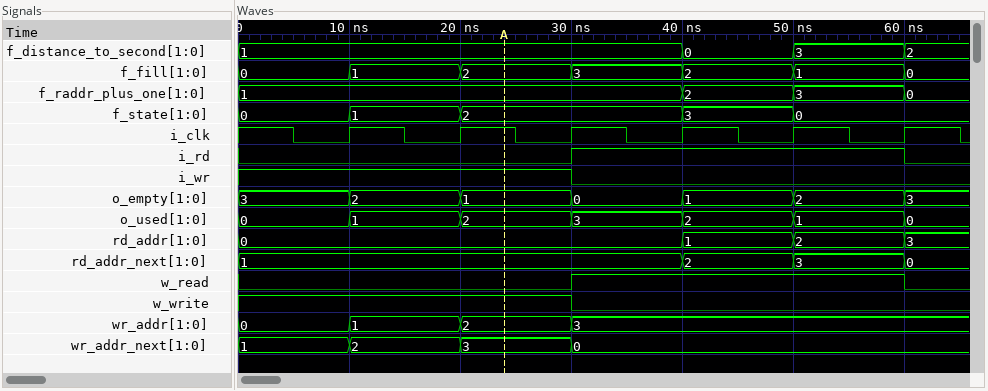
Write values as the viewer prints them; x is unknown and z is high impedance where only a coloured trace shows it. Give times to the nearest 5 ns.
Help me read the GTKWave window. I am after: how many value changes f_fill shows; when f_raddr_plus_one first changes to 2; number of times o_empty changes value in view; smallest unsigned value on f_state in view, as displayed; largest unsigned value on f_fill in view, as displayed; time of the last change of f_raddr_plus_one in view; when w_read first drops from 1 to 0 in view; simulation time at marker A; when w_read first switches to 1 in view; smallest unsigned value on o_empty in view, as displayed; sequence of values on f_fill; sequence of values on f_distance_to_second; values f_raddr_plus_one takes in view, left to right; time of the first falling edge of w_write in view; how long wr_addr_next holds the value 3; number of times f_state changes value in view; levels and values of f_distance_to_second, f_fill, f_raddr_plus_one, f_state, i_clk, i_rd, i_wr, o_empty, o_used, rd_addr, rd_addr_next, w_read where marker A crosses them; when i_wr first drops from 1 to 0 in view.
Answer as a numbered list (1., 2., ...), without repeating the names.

1. 6
2. 40 ns
3. 6
4. 0
5. 3
6. 60 ns
7. 60 ns
8. 25 ns
9. 30 ns
10. 0
11. 0, 1, 2, 3, 2, 1, 0
12. 1, 0, 3, 2
13. 1, 2, 3, 0
14. 30 ns
15. 10 ns
16. 4
17. f_distance_to_second=1, f_fill=2, f_raddr_plus_one=1, f_state=2, i_clk=1, i_rd=0, i_wr=1, o_empty=1, o_used=2, rd_addr=0, rd_addr_next=1, w_read=0
18. 30 ns
